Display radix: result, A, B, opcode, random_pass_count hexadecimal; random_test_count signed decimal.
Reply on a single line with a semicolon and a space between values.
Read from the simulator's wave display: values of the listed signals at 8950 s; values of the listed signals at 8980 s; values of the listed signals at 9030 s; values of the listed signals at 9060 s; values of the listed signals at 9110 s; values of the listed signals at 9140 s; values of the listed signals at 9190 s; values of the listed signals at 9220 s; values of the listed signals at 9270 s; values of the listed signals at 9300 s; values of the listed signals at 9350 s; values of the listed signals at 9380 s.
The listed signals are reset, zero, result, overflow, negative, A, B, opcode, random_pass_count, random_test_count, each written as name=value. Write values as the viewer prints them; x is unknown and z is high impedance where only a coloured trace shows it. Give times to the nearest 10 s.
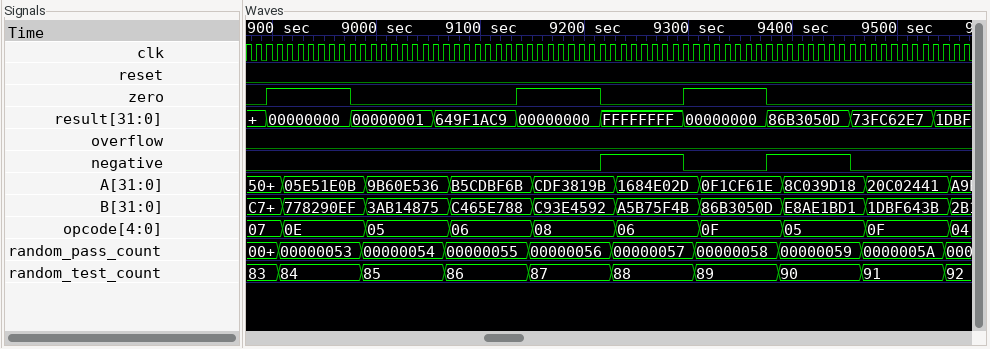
reset=0, zero=1, result=00000000, overflow=0, negative=0, A=05E51E0B, B=778290EF, opcode=0E, random_pass_count=00000053, random_test_count=84; reset=0, zero=0, result=00000001, overflow=0, negative=0, A=05E51E0B, B=778290EF, opcode=0E, random_pass_count=00000053, random_test_count=84; reset=0, zero=0, result=00000001, overflow=0, negative=0, A=9B60E536, B=3AB14875, opcode=05, random_pass_count=00000054, random_test_count=85; reset=0, zero=0, result=649F1AC9, overflow=0, negative=0, A=9B60E536, B=3AB14875, opcode=05, random_pass_count=00000054, random_test_count=85; reset=0, zero=0, result=649F1AC9, overflow=0, negative=0, A=B5CDBF6B, B=C465E788, opcode=06, random_pass_count=00000055, random_test_count=86; reset=0, zero=1, result=00000000, overflow=0, negative=0, A=B5CDBF6B, B=C465E788, opcode=06, random_pass_count=00000055, random_test_count=86; reset=0, zero=1, result=00000000, overflow=0, negative=0, A=CDF3819B, B=C93E4592, opcode=08, random_pass_count=00000056, random_test_count=87; reset=0, zero=0, result=FFFFFFFF, overflow=0, negative=1, A=CDF3819B, B=C93E4592, opcode=08, random_pass_count=00000056, random_test_count=87; reset=0, zero=0, result=FFFFFFFF, overflow=0, negative=1, A=1684E02D, B=A5B75F4B, opcode=06, random_pass_count=00000057, random_test_count=88; reset=0, zero=1, result=00000000, overflow=0, negative=0, A=1684E02D, B=A5B75F4B, opcode=06, random_pass_count=00000057, random_test_count=88; reset=0, zero=1, result=00000000, overflow=0, negative=0, A=0F1CF61E, B=86B3050D, opcode=0F, random_pass_count=00000058, random_test_count=89; reset=0, zero=0, result=86B3050D, overflow=0, negative=1, A=0F1CF61E, B=86B3050D, opcode=0F, random_pass_count=00000058, random_test_count=89
